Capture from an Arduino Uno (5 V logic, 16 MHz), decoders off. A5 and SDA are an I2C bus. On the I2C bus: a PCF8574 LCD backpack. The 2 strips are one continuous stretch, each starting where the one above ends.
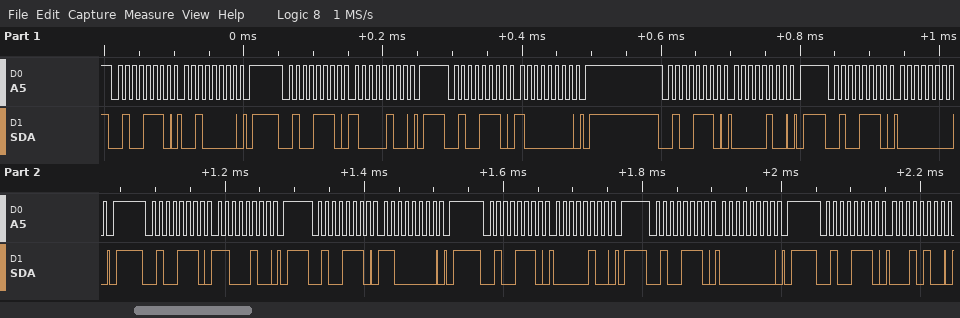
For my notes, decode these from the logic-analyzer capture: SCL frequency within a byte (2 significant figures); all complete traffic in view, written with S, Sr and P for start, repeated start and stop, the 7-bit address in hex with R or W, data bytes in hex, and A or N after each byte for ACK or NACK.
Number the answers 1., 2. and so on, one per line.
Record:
1. 100 kHz
2. S 27W A 20 A P S 27W A 84 A P S 27W A 80 A P S 27W A 04 A P S 27W A 00 A P S 27W A C4 A P S 27W A C0 A P S 27W A 04 A P S 27W A 00 A P S 27W A 14 A
